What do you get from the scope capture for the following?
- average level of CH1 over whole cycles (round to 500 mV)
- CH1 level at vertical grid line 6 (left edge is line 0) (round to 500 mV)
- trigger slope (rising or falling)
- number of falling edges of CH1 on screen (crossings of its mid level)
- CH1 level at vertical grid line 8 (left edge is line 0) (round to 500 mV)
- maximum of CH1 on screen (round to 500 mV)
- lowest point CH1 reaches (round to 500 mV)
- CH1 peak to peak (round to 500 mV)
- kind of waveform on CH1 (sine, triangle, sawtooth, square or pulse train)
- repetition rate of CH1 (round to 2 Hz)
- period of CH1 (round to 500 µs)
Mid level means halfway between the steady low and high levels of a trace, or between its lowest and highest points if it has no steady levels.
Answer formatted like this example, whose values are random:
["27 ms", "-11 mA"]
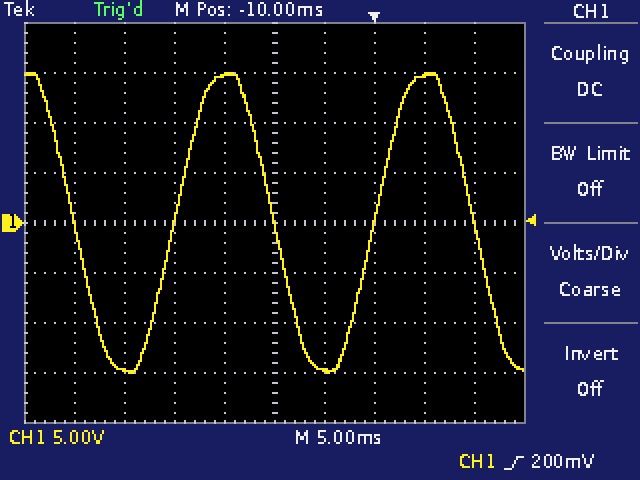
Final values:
["0.0 V", "-15.0 V", "rising", "3", "15.0 V", "15.0 V", "-15.0 V", "30.0 V", "sine", "50 Hz", "20.0 ms"]
